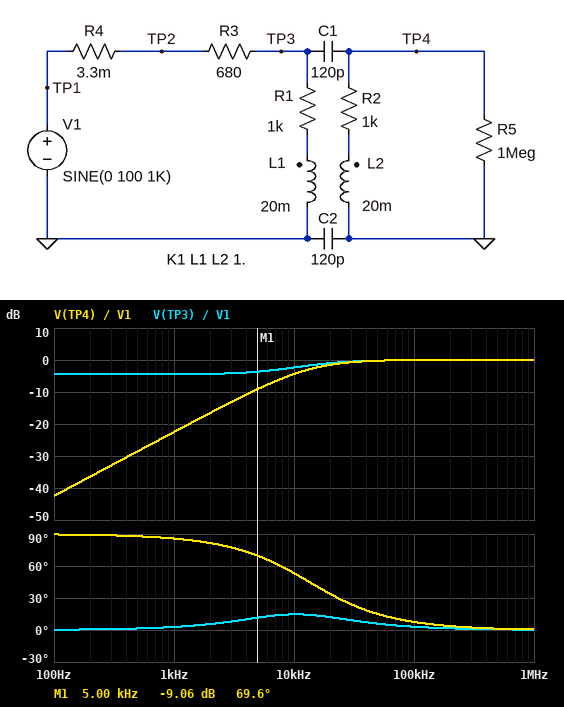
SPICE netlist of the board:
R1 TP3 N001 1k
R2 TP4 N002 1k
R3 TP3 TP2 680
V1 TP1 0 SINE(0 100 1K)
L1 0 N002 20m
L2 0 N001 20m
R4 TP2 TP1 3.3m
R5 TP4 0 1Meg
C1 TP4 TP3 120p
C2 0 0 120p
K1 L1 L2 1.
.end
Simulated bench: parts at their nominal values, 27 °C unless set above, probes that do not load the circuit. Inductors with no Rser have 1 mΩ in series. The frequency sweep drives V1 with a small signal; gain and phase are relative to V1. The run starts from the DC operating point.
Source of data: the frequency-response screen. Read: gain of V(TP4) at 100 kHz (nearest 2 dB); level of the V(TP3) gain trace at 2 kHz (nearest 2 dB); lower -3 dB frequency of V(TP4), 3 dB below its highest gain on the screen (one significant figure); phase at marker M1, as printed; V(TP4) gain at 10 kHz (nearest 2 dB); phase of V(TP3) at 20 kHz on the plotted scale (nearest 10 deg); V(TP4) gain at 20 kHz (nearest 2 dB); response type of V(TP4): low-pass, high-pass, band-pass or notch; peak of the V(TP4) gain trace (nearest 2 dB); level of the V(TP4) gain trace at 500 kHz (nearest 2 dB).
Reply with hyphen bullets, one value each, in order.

- 0 dB
- -4 dB
- 10 kHz
- 69.6 deg
- -4 dB
- 10 deg
- -2 dB
- high-pass
- 0 dB
- 0 dB
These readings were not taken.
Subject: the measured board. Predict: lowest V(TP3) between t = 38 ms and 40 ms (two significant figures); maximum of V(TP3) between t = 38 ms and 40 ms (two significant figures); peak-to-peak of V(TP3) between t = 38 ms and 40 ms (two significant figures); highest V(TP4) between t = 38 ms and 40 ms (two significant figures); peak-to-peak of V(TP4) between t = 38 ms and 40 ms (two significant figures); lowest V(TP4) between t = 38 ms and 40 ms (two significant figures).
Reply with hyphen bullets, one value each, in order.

- -60 V
- 60 V
- 120 V
- 7.5 V
- 15 V
- -7.5 V
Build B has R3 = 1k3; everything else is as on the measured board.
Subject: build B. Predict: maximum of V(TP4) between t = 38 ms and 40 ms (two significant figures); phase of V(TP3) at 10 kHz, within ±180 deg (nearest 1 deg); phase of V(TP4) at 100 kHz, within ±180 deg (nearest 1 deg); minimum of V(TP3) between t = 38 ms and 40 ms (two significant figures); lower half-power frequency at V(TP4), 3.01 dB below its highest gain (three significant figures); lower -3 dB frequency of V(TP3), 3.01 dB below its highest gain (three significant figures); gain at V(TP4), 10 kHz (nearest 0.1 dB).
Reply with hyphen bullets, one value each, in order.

- 5.5 V
- 23 deg
- 10 deg
- -44 V
- 18.2 kHz
- 14.5 kHz
- -6.3 dB
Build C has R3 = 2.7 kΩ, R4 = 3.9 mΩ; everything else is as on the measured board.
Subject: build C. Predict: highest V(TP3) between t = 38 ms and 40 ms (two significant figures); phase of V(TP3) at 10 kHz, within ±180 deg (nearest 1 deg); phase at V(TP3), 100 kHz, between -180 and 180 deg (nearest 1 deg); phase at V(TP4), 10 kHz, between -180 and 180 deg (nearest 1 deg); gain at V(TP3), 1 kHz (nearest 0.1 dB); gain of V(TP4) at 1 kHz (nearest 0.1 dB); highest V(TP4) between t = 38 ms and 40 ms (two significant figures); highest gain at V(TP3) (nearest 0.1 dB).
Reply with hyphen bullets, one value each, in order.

- 27 V
- 33 deg
- 12 deg
- 71 deg
- -11.3 dB
- -29.3 dB
- 3.4 V
- 0 dB
